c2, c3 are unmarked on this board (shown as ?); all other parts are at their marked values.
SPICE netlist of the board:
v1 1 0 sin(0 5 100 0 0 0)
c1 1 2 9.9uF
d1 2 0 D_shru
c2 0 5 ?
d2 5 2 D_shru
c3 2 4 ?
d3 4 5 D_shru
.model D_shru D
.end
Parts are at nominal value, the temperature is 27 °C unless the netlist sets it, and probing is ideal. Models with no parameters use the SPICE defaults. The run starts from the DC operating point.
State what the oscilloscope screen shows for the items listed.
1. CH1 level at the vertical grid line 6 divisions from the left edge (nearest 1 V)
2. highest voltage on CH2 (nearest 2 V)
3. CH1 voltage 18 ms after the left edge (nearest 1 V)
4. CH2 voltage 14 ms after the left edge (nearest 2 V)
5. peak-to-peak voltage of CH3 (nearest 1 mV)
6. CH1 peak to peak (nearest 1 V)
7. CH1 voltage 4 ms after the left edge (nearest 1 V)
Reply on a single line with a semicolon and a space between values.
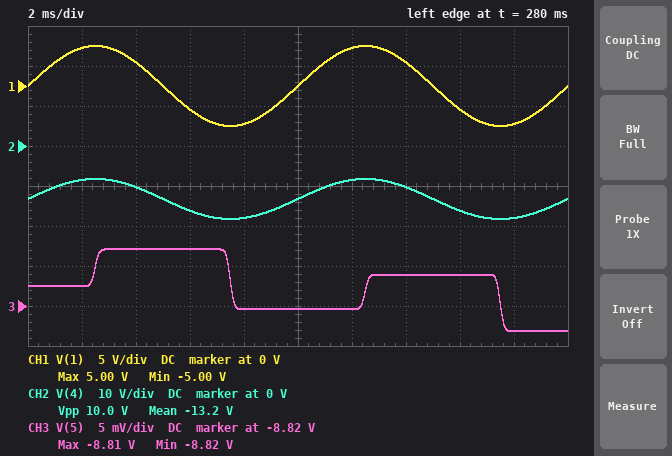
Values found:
5 V; -8 V; -5 V; -10 V; 10 mV; 10 V; 3 V
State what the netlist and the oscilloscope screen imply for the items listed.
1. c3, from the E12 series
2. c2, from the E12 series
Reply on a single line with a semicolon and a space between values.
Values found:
4.7 µF; 3.3 µF
